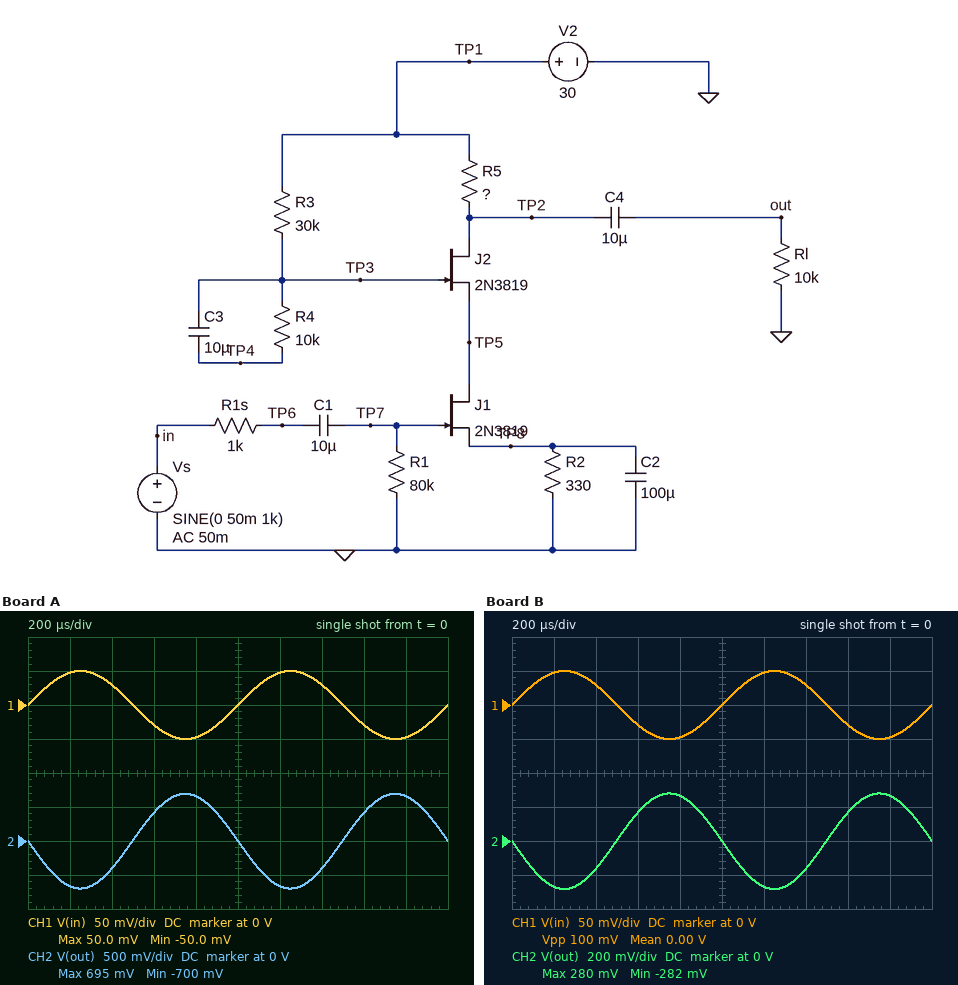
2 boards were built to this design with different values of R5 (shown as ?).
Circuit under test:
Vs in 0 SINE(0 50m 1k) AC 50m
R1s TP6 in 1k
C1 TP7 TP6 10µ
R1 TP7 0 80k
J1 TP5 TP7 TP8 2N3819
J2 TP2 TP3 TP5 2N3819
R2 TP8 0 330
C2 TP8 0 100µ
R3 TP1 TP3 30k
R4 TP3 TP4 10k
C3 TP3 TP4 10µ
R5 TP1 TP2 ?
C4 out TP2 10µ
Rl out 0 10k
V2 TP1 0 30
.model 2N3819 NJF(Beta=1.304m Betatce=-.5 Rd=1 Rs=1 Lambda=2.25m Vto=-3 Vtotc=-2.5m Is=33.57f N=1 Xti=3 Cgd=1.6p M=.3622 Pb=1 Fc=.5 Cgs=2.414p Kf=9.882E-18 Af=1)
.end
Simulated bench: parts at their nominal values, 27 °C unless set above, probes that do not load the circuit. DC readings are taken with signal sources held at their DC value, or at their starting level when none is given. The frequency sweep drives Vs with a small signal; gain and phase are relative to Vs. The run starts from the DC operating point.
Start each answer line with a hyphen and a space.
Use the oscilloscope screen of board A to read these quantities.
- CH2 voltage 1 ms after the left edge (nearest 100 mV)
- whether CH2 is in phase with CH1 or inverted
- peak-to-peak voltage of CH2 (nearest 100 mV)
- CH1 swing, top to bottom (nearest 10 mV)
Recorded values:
- 0 V
- inverted
- 1.4 V
- 100 mV
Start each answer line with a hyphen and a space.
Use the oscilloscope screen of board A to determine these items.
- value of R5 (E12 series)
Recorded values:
- 5.6 kΩ
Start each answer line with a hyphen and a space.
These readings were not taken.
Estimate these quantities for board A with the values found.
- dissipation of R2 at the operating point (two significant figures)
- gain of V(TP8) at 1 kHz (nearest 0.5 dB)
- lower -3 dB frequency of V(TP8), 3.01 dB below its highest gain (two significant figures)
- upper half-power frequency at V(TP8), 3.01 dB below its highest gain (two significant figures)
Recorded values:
- 5.0 mW
- -43.0 dB
- 190 mHz
- 12 Hz
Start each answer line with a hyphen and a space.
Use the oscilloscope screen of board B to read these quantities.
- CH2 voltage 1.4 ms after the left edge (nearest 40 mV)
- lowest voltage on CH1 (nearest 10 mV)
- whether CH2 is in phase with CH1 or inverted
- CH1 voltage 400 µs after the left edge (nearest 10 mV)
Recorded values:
- -160 mV
- -50 mV
- inverted
- 30 mV
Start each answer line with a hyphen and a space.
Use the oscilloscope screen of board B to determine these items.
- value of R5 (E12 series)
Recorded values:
- 1.5 kΩ
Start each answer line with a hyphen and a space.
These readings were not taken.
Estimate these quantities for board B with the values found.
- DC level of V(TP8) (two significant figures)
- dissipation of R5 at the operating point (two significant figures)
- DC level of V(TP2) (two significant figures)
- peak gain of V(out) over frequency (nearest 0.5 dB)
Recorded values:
- 1.3 V
- 21 mW
- 24 V
- 15.0 dB
